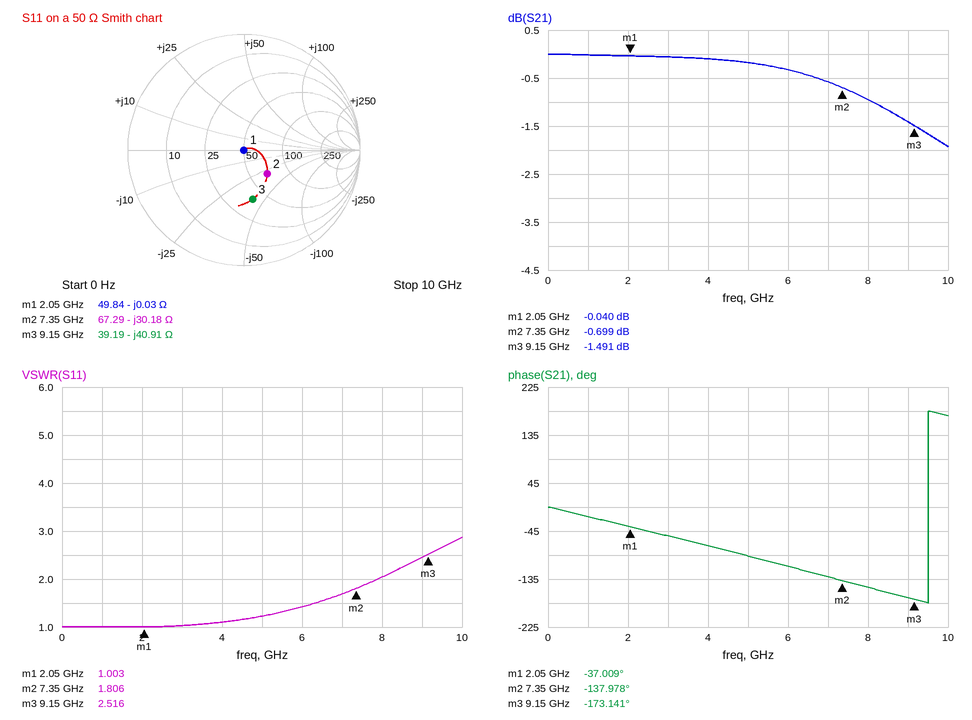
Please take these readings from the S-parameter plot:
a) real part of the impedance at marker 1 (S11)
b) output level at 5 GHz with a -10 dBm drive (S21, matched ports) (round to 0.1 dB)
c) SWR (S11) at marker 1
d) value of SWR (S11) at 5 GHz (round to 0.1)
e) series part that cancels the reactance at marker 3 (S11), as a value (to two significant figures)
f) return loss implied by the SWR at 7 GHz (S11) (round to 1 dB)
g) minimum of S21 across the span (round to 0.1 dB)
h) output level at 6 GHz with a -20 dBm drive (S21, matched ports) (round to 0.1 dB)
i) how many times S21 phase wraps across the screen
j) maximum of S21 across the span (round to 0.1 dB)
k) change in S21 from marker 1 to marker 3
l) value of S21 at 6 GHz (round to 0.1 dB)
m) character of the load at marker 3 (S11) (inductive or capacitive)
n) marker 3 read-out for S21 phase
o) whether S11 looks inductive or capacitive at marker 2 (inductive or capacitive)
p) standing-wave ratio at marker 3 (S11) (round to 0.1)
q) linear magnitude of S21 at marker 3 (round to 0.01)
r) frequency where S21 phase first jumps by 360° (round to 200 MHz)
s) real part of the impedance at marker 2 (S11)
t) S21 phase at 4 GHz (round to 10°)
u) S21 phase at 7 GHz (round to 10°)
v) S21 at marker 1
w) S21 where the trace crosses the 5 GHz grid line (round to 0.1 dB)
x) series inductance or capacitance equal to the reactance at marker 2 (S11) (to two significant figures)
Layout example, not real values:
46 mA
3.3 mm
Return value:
49.84 Ω
-10.2 dBm
1.003
1.2
710 pH
12 dB
-1.9 dB
-20.3 dBm
1
0.0 dB
-1.451 dB
-0.3 dB
capacitive
-173.141°
capacitive
2.5
0.84
9.6 GHz
67.29 Ω
-70°
-130°
-0.040 dB
-0.2 dB
720 fF
